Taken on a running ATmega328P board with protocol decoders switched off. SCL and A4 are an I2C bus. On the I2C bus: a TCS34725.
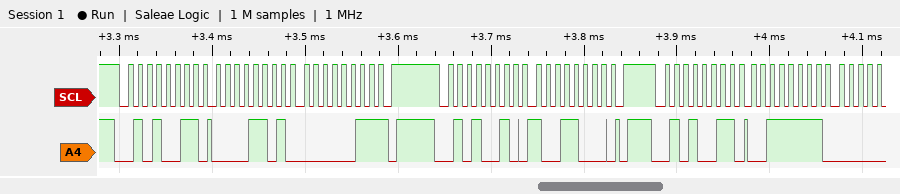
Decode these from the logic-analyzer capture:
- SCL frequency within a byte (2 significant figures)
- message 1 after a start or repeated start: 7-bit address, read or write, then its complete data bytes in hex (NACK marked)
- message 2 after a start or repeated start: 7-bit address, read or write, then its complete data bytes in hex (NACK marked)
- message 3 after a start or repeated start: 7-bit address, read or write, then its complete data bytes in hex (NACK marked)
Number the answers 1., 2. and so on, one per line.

1. 100 kHz
2. 0x29 read: 0D 03 NACK
3. 0x29 write: 98
4. 0x29 read: 3F
